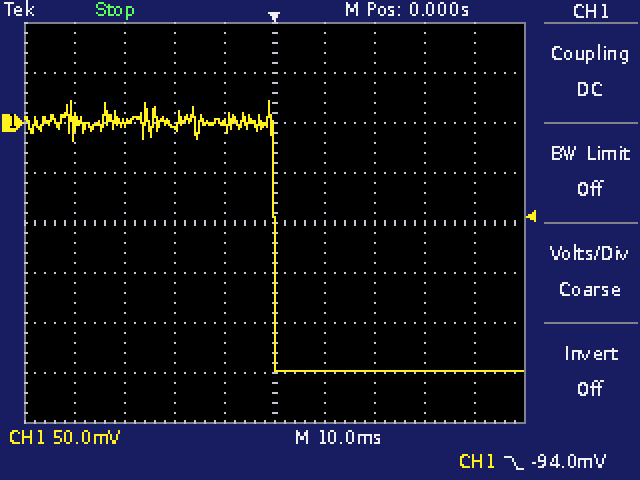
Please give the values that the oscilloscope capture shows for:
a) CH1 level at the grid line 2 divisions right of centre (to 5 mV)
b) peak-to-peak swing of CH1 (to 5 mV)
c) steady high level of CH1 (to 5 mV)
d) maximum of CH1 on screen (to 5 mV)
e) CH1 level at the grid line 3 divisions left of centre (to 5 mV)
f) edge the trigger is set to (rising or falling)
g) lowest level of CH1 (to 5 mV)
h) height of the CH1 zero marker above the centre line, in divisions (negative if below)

-250 mV
270 mV
0 mV
20 mV
0 mV
falling
-250 mV
+2.0 div
